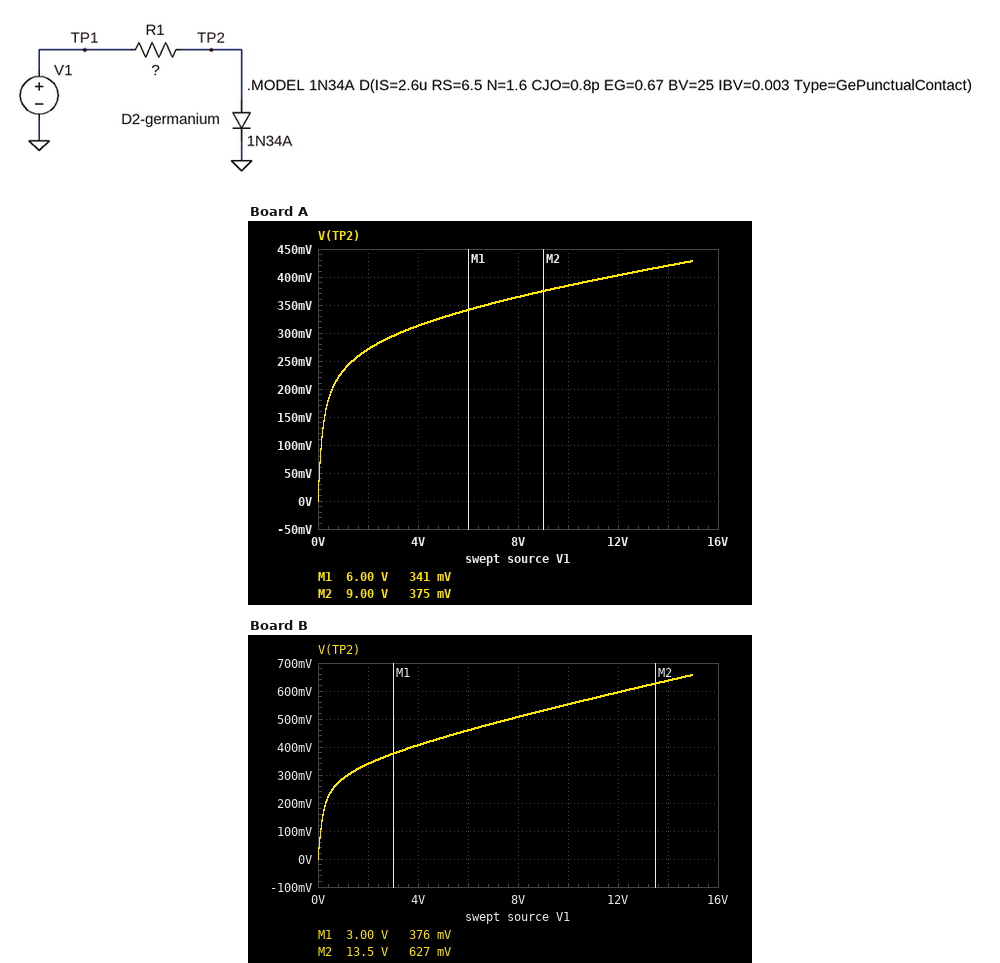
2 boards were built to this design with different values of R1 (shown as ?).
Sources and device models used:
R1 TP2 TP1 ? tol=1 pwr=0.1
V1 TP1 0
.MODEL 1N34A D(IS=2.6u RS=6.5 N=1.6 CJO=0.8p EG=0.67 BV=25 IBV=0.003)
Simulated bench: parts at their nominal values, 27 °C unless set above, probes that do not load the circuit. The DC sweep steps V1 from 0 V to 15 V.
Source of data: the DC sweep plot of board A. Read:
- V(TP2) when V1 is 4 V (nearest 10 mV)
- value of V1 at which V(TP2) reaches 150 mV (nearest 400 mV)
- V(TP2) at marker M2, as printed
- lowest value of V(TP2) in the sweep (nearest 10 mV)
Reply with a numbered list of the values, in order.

1. 310 mV
2. 400 mV
3. 375 mV
4. 0 V
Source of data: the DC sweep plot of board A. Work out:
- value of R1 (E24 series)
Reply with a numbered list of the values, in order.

1. 1.2 kΩ
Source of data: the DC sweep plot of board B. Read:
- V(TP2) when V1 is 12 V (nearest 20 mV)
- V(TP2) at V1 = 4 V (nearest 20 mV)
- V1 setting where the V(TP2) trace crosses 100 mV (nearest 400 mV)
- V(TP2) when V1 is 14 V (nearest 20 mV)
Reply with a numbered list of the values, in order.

1. 600 mV
2. 400 mV
3. 0 V
4. 640 mV
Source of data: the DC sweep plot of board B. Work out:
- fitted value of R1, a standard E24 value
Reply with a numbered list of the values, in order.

1. 360 Ω
